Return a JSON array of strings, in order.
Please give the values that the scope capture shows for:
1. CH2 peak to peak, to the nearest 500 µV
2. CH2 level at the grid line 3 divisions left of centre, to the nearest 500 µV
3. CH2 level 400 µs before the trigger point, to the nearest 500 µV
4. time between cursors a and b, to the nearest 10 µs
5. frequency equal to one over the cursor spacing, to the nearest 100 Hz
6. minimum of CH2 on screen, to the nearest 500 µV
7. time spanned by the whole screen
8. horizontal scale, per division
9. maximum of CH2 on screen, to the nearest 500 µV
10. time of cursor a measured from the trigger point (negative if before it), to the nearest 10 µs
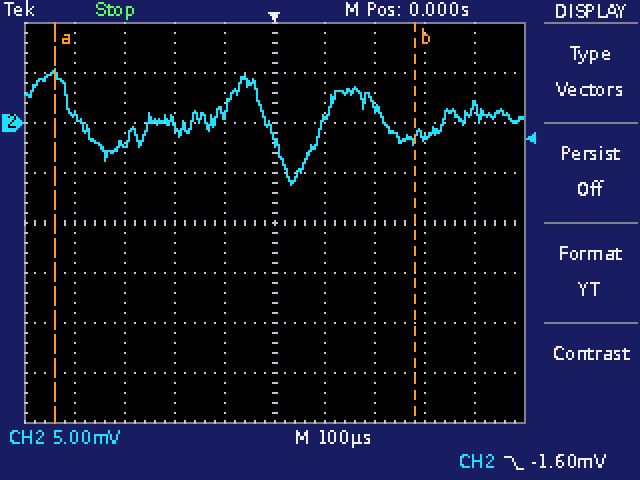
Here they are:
["11.5 mV", "-2.0 mV", "500 µV", "720 µs", "1.4 kHz", "-6.0 mV", "1 ms", "100 µs", "5.5 mV", "-440 µs"]
